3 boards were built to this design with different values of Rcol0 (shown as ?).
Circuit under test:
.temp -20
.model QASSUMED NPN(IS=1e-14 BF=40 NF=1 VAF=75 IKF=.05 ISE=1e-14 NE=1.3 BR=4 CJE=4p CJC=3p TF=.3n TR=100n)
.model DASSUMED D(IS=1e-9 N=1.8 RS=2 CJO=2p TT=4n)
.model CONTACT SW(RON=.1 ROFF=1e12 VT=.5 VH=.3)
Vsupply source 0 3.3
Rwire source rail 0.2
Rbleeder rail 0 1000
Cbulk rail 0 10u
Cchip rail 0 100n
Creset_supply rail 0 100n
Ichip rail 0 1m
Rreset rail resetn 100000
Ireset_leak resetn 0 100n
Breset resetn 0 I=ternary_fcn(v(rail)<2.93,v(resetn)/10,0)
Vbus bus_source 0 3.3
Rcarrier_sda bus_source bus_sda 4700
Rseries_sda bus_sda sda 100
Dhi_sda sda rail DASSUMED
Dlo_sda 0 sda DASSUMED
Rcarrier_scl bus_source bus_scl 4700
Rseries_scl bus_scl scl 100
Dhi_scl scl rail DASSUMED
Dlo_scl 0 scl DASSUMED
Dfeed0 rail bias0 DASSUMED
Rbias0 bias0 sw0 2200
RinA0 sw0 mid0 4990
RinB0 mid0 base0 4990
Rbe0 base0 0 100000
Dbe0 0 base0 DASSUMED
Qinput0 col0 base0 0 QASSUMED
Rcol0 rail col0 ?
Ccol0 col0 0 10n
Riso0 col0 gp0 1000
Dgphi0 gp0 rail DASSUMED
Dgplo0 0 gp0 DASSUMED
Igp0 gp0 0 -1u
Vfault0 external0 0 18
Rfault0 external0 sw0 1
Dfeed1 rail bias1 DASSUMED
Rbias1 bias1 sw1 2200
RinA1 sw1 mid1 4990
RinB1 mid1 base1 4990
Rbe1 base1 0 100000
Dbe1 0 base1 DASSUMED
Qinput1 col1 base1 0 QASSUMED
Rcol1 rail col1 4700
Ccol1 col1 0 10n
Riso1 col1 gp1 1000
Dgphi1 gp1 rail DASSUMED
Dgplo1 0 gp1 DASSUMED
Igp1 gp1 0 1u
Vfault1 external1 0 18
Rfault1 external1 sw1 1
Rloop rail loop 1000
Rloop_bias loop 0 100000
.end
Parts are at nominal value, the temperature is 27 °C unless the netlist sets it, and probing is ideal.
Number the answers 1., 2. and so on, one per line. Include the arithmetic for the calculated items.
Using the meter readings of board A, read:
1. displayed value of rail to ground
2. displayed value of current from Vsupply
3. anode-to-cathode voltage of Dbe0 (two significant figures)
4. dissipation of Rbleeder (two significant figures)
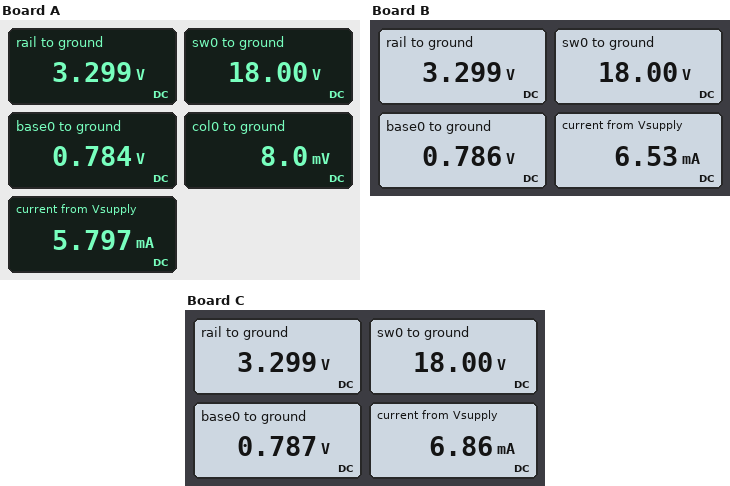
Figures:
1. 3.299 V
2. 5.797 mA
3. 0 V - 784 mV = -780 mV
4. (3.299 V)^2 / 1 kΩ = 11 mW
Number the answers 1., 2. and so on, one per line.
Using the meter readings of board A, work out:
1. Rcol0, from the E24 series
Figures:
1. 4.3 kΩ
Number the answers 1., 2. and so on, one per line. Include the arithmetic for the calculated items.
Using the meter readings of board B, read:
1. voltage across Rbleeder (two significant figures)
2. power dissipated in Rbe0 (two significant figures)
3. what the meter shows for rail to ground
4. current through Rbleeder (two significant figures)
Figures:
1. 3.299 V = 3.3 V
2. (786 mV)^2 / 100 kΩ = 6.2 µW
3. 3.299 V
4. (3.299 V) / 1 kΩ = 3.3 mA
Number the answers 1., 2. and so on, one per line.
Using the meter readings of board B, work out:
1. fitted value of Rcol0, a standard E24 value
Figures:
1. 2.2 kΩ
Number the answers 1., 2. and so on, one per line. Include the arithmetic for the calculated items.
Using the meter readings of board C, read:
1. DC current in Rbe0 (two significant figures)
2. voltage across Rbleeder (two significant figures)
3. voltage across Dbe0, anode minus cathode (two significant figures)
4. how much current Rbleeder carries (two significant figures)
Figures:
1. (787 mV) / 100 kΩ = 7.9 µA
2. 3.299 V = 3.3 V
3. 0 V - 787 mV = -790 mV
4. (3.299 V) / 1 kΩ = 3.3 mA
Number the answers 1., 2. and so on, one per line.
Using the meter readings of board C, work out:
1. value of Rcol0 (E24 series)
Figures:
1. 1.8 kΩ
